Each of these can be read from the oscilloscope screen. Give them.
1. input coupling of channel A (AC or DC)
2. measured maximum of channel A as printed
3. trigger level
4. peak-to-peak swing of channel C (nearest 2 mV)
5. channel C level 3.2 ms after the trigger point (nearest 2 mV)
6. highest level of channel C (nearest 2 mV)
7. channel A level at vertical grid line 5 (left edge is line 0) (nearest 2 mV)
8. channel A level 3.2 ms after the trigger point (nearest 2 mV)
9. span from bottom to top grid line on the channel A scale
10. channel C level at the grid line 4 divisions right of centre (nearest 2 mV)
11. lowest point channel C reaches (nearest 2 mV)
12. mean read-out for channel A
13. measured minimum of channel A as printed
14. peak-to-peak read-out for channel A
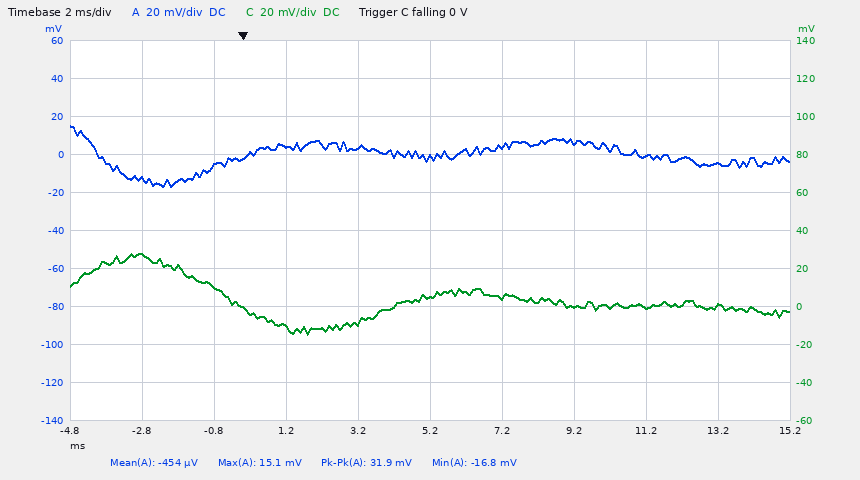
DC
15.1 mV
0 V
42 mV
-8 mV
28 mV
-2 mV
4 mV
200 mV
0 mV
-14 mV
-454 µV
-16.8 mV
31.9 mV
